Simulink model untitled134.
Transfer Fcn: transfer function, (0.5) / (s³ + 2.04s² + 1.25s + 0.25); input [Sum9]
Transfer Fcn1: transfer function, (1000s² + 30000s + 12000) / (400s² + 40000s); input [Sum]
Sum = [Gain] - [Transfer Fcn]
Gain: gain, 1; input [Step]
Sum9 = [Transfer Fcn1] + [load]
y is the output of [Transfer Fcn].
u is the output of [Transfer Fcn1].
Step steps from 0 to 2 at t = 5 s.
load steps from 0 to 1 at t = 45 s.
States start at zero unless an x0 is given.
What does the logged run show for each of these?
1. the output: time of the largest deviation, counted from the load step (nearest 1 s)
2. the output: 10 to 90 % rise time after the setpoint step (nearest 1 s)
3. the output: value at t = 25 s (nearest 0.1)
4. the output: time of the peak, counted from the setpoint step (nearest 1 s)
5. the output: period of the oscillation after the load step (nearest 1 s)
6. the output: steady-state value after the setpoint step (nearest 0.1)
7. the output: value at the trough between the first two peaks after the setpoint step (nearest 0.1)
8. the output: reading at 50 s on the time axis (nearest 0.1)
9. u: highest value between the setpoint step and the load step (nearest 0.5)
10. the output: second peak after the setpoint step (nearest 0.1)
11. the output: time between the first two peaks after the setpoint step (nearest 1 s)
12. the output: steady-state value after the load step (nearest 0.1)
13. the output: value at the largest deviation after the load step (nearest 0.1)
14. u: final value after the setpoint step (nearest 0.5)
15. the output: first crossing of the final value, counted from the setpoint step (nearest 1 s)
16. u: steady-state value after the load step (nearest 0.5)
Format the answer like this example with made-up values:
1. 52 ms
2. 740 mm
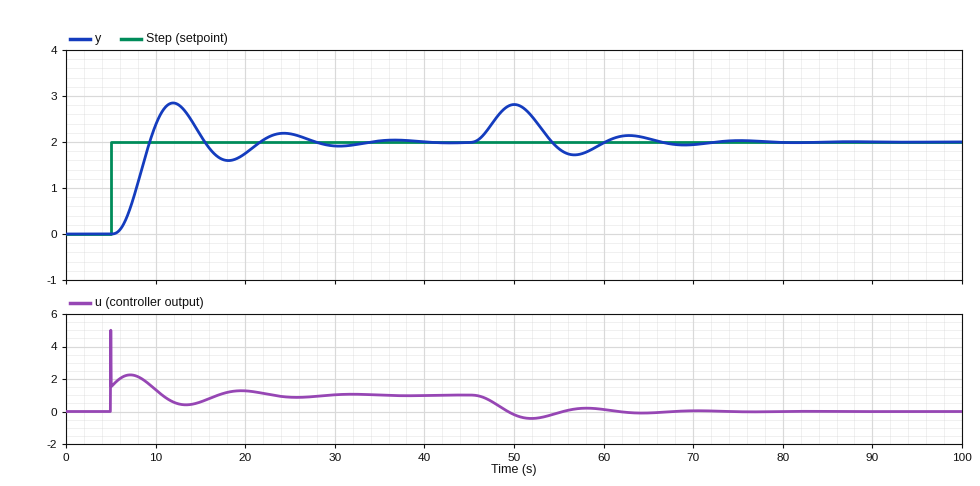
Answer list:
1. 5 s
2. 3 s
3. 2.2
4. 7 s
5. 13 s
6. 2.0
7. 1.6
8. 2.8
9. 5.0
10. 2.2
11. 12 s
12. 2.0
13. 2.8
14. 1.0
15. 4 s
16. 0.0
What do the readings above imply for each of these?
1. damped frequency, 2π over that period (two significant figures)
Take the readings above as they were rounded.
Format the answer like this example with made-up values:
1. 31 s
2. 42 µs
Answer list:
1. 0.52 rad/s
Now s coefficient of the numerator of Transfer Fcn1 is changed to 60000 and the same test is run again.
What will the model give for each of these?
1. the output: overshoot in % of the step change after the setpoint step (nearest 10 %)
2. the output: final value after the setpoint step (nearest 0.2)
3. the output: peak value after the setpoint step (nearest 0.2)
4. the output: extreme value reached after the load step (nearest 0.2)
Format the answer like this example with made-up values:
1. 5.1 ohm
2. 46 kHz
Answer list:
1. 40 %
2. 2.0
3. 2.8
4. 2.6
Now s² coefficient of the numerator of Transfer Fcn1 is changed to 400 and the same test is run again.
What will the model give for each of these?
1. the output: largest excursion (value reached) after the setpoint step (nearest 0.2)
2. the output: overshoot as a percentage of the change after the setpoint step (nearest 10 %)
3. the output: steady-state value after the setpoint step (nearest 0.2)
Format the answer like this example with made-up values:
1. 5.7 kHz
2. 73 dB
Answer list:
1. 2.8
2. 40 %
3. 2.0
